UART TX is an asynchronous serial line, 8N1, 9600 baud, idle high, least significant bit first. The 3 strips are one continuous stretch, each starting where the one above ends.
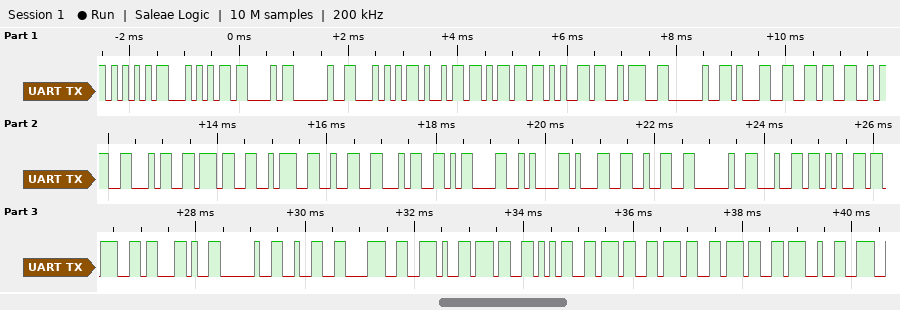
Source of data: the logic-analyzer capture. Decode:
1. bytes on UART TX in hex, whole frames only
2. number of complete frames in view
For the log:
55 54 43 20 54 69 6D 65 3A 20 31 36 3A 34 37 3A 32 34 0D 0A 31 32 20 64 65 67 2C 20 32 38 2E 37 35 37 37 37 27
37
